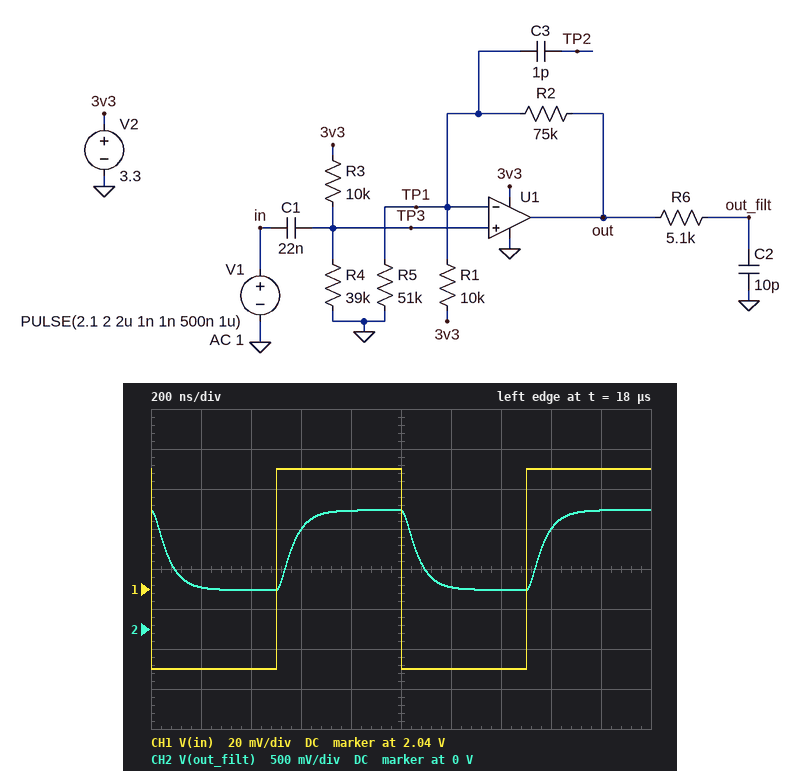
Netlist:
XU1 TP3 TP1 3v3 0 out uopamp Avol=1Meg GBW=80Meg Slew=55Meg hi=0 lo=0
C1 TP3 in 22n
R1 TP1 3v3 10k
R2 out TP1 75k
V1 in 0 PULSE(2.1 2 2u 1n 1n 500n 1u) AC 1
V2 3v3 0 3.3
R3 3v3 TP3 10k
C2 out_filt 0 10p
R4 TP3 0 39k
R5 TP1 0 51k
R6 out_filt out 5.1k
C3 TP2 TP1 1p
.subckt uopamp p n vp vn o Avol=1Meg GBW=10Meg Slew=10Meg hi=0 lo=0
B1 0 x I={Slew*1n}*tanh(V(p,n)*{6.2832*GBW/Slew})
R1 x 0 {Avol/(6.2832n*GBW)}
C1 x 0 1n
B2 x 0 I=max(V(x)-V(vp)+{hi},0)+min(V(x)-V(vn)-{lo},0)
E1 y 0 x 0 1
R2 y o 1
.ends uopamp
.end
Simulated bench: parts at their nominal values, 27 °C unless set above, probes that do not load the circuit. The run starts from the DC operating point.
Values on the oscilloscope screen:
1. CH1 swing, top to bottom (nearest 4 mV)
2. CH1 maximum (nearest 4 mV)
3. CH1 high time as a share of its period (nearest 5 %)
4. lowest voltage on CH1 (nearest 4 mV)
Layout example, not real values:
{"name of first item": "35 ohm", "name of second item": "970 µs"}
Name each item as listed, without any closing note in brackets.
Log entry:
{"CH1 swing, top to bottom": "100 mV", "CH1 maximum": "2.100 V", "CH1 high time as a share of its period": "50 %", "lowest voltage on CH1": "2.000 V"}
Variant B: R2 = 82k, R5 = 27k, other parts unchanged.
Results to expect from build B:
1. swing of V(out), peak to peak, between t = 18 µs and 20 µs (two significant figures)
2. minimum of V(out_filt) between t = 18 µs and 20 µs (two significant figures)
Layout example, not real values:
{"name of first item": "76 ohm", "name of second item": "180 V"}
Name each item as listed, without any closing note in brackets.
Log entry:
{"swing of V(out), peak to peak, between t = 18 µs and 20 µs": "25 mV", "minimum of V(out_filt) between t = 18 µs and 20 µs": "3.3 V"}
